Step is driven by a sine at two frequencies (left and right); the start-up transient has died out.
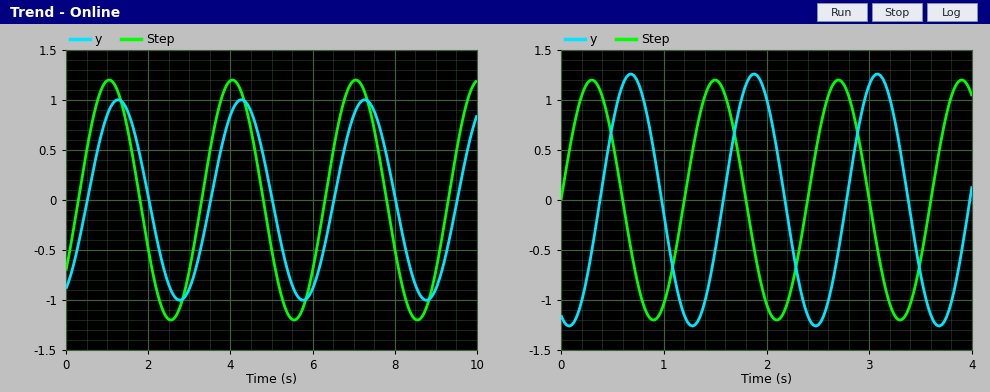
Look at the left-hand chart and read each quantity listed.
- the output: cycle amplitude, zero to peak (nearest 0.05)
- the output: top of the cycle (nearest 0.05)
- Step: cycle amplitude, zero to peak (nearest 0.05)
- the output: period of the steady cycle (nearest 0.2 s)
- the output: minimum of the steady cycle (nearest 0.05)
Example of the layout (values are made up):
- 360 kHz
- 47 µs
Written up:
- 1.00
- 1.00
- 1.20
- 3.0 s
- -1.00
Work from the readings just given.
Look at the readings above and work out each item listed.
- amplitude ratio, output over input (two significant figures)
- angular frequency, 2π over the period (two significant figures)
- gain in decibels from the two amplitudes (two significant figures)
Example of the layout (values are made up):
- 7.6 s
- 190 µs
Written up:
- 0.83
- 2.1 rad/s
- -1.6 dB
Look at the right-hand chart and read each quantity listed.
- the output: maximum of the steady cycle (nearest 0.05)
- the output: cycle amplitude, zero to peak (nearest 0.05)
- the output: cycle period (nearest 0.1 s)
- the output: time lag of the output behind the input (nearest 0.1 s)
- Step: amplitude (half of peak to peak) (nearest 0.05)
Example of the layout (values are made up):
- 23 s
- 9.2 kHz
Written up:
- 1.25
- 1.25
- 1.2 s
- 0.4 s
- 1.20
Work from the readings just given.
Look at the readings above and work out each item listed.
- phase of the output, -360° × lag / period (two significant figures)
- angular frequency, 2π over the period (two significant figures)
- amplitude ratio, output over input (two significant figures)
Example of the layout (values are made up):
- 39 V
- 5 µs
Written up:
- -120°
- 5.2 rad/s
- 1.0
